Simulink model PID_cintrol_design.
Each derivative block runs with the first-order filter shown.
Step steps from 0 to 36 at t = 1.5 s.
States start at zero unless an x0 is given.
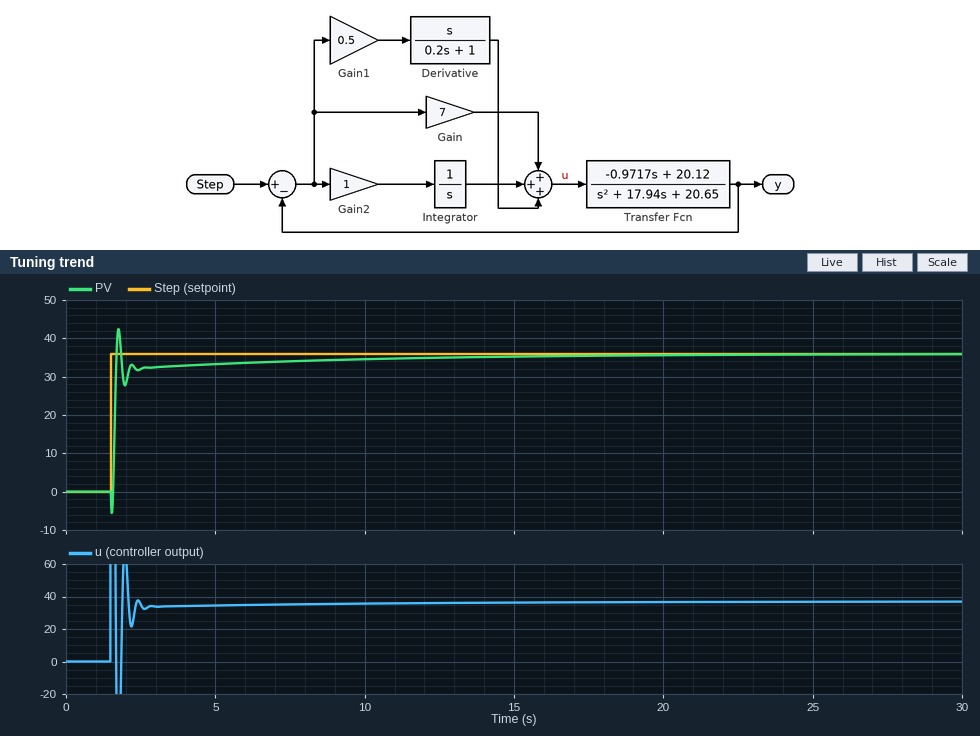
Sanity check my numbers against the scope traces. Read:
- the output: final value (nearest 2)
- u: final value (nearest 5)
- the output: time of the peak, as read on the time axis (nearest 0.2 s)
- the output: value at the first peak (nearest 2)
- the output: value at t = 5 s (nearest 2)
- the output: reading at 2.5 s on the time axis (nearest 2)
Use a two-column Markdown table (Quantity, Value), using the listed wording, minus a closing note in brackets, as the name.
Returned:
| Quantity | Value |
|---|---|
| the output: final value | 36 |
| u: final value | 35 |
| the output: time of the peak, as read on the time axis | 1.8 s |
| the output: value at the first peak | 42 |
| the output: value at t = 5 s | 34 |
| the output: reading at 2.5 s on the time axis | 32 |
